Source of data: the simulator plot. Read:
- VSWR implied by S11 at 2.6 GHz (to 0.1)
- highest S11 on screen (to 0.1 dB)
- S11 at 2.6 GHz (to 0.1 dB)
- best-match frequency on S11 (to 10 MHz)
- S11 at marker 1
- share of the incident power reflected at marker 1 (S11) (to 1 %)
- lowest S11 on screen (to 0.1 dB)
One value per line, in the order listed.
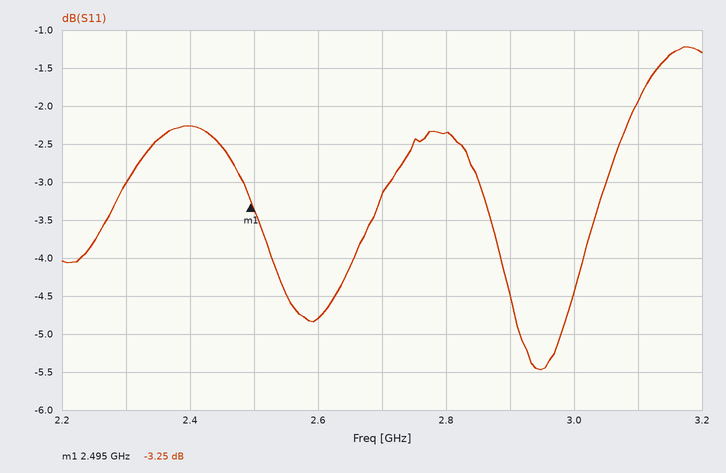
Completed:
3.7
-1.2 dB
-4.8 dB
2.95 GHz
-3.25 dB
47 %
-5.5 dB
